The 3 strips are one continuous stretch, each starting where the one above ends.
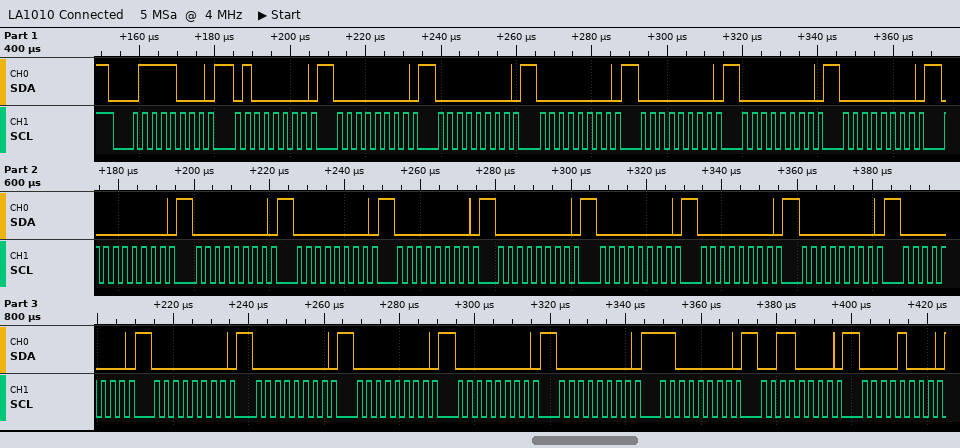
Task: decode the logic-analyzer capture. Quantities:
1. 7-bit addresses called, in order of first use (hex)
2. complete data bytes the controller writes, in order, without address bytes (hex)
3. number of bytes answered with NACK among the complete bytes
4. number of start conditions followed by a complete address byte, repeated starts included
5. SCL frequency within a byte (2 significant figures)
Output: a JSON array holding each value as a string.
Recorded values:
["0x3C", "40 00 00 00 00 00 00 00 00 00 00 00 00 00 00 00 00 00 00 00 00 C0 30 08", "0", "1", "400 kHz"]
